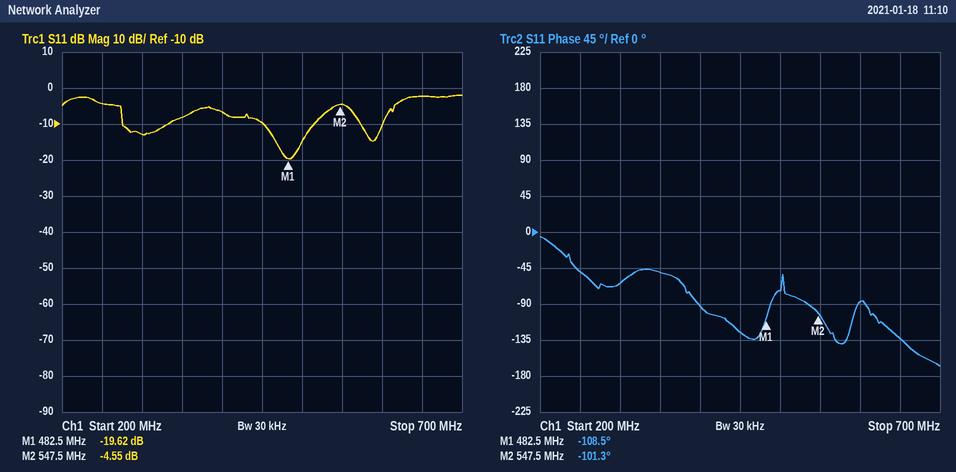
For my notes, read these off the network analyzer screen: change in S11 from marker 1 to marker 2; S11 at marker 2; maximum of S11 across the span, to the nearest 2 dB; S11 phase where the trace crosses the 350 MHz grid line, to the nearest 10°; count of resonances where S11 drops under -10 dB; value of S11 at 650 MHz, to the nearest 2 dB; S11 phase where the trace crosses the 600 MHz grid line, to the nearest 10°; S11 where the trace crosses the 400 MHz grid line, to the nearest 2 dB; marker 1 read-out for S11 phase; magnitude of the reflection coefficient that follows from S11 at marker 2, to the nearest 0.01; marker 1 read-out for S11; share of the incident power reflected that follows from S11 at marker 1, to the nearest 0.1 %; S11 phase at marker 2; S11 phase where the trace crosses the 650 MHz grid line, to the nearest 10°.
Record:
15.07 dB
-4.55 dB
-2 dB
-50°
3
-2 dB
-90°
-6 dB
-108.5°
0.59
-19.62 dB
1.1 %
-101.3°
-130°
